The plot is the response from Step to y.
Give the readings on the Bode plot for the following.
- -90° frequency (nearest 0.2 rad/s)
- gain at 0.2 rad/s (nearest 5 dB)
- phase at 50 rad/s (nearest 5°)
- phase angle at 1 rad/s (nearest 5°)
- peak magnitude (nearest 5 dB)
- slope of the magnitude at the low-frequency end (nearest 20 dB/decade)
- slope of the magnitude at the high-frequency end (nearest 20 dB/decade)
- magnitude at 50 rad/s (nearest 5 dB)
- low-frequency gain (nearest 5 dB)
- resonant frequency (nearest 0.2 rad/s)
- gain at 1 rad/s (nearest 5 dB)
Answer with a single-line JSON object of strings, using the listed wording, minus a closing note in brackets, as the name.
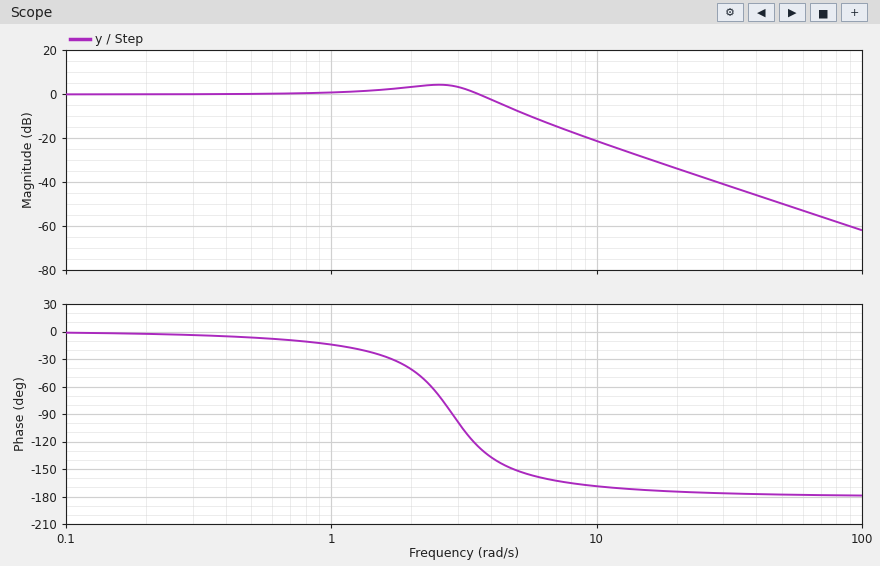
{"-90° frequency": "2.8 rad/s", "gain at 0.2 rad/s": "0 dB", "phase at 50 rad/s": "-180°", "phase angle at 1 rad/s": "-15°", "peak magnitude": "5 dB", "slope of the magnitude at the low-frequency end": "0 dB/decade", "slope of the magnitude at the high-frequency end": "-40 dB/decade", "magnitude at 50 rad/s": "-50 dB", "low-frequency gain": "0 dB", "resonant frequency": "2.6 rad/s", "gain at 1 rad/s": "0 dB"}
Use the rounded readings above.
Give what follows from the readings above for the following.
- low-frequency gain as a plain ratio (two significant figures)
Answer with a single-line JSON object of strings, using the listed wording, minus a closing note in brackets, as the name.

{"low-frequency gain as a plain ratio": "1.0"}
